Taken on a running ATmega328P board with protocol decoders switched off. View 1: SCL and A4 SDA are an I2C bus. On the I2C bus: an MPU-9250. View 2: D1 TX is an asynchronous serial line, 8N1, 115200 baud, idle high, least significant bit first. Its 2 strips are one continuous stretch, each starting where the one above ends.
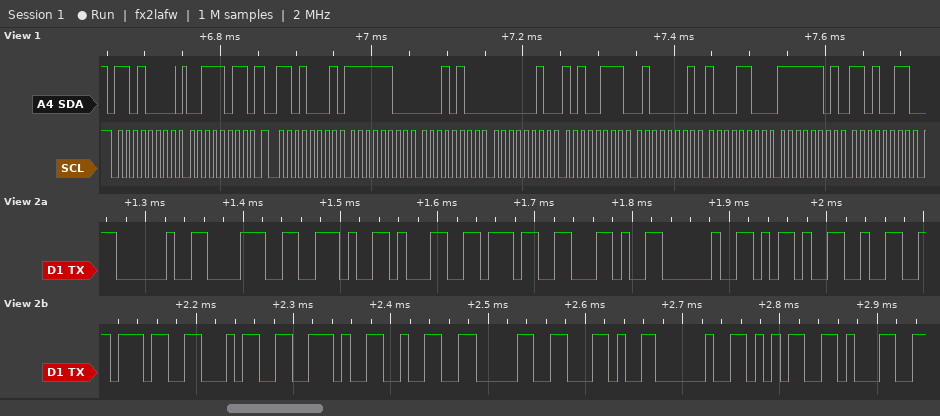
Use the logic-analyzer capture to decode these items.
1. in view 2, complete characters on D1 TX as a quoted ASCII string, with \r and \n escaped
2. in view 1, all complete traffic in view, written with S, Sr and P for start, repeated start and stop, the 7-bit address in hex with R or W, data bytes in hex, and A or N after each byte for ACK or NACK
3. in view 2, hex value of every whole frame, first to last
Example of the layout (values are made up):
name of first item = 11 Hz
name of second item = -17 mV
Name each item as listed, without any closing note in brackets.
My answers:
in view 2, complete characters on D1 TX as a quoted ASCII string, with \r and \n escaped = " 8.17, -274.20, 51"
in view 1, all complete traffic in view, written with S, Sr and P for start, repeated start and stop, the 7-bit address in hex with R or W, data bytes in hex, and A or N after each byte for ACK or NACK = S 68W A 3B A Sr 68R A FC A 14 A 02 A A7 A 41 A 8C A FD A D3 A
in view 2, hex value of every whole frame, first to last = 0x20 0x38 0x2E 0x31 0x37 0x2C 0x20 0x2D 0x32 0x37 0x34 0x2E 0x32 0x30 0x2C 0x20 0x35 0x31
